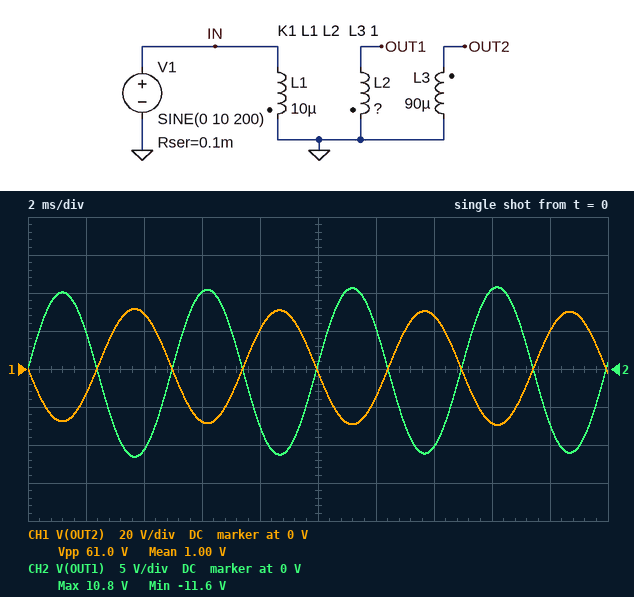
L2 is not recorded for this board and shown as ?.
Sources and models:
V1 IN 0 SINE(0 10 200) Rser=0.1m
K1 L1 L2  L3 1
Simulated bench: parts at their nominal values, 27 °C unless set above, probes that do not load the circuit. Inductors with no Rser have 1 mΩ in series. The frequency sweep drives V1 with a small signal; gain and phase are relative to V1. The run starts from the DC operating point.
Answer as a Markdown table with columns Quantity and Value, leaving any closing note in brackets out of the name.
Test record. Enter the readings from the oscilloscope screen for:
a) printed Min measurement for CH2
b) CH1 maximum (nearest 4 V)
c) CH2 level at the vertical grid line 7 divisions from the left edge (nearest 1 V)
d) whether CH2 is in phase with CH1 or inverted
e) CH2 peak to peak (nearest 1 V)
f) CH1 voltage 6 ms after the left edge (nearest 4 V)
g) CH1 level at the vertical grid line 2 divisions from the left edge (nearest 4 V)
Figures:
| Quantity | Value |
|---|---|
| printed Min measurement for CH2 | -11.6 V |
| CH1 maximum | 32 V |
| CH2 level at the vertical grid line 7 divisions from the left edge | -10 V |
| whether CH2 is in phase with CH1 or inverted | inverted |
| CH2 peak to peak | 22 V |
| CH1 voltage 6 ms after the left edge | -28 V |
| CH1 level at the vertical grid line 2 divisions from the left edge | 28 V |
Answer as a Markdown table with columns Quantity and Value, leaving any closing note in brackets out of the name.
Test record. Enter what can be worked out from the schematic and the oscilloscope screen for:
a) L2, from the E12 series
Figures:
| Quantity | Value |
|---|---|
| L2, from the E12 series | 12 µH |
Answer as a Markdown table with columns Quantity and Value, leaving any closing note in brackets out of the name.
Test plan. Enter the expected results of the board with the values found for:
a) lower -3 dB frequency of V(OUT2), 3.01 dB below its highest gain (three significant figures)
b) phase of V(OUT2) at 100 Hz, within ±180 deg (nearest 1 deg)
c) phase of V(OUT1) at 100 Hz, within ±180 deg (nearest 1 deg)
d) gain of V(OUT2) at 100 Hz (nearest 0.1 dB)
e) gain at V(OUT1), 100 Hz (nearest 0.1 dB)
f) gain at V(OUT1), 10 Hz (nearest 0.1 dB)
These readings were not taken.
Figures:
| Quantity | Value |
|---|---|
| lower -3 dB frequency of V(OUT2), 3.01 dB below its highest gain | 17.5 Hz |
| phase of V(OUT2) at 100 Hz, within ±180 deg | -170 deg |
| phase of V(OUT1) at 100 Hz, within ±180 deg | 10 deg |
| gain of V(OUT2) at 100 Hz | 9.4 dB |
| gain at V(OUT1), 100 Hz | 0.7 dB |
| gain at V(OUT1), 10 Hz | -5.3 dB |
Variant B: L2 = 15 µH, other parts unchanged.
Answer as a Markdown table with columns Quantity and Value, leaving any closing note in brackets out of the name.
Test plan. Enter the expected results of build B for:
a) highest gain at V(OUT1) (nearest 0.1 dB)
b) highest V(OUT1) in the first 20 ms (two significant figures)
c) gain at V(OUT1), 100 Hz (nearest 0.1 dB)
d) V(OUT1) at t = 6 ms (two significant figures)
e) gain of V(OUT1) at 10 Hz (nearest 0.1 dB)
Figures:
| Quantity | Value |
|---|---|
| highest gain at V(OUT1) | 1.8 dB |
| highest V(OUT1) in the first 20 ms | 12 V |
| gain at V(OUT1), 100 Hz | 1.6 dB |
| V(OUT1) at t = 6 ms | 11 V |
| gain of V(OUT1) at 10 Hz | -4.3 dB |
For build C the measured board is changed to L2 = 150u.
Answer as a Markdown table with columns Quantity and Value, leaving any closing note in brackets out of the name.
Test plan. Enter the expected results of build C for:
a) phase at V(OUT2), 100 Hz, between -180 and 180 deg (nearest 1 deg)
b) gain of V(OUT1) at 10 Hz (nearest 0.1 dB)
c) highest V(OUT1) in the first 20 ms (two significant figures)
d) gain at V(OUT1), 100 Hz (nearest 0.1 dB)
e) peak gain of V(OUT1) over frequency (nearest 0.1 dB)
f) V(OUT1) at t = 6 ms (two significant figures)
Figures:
| Quantity | Value |
|---|---|
| phase at V(OUT2), 100 Hz, between -180 and 180 deg | -170 deg |
| gain of V(OUT1) at 10 Hz | 5.7 dB |
| highest V(OUT1) in the first 20 ms | 38 V |
| gain at V(OUT1), 100 Hz | 11.6 dB |
| peak gain of V(OUT1) over frequency | 11.8 dB |
| V(OUT1) at t = 6 ms | 36 V |
